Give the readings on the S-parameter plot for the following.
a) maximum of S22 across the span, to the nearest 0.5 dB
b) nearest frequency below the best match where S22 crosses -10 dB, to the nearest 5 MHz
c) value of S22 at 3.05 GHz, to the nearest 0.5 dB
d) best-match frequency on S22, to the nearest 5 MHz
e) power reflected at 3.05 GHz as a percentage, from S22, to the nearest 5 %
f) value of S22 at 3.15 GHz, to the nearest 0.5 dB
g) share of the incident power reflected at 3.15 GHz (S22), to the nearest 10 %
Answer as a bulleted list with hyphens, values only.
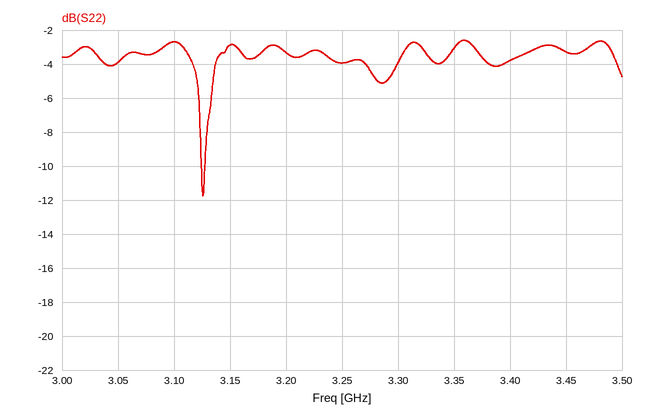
- -2.5 dB
- 3.125 GHz
- -4.0 dB
- 3.125 GHz
- 40 %
- -3.0 dB
- 50 %
